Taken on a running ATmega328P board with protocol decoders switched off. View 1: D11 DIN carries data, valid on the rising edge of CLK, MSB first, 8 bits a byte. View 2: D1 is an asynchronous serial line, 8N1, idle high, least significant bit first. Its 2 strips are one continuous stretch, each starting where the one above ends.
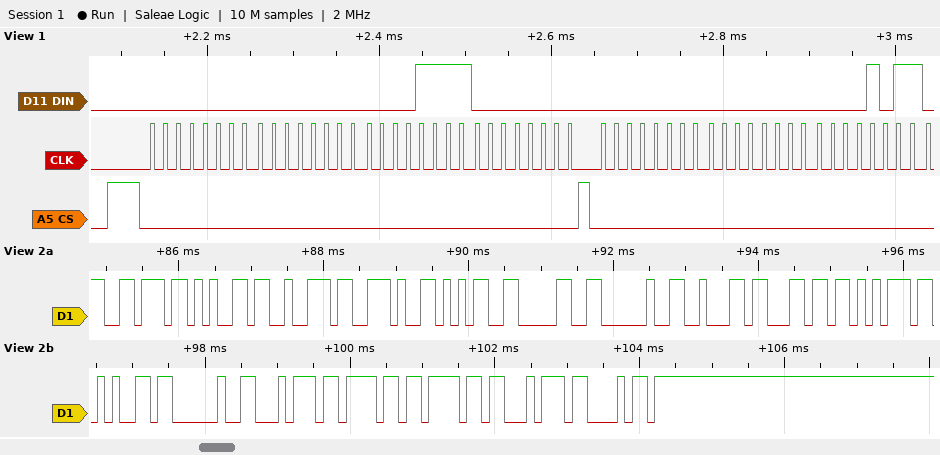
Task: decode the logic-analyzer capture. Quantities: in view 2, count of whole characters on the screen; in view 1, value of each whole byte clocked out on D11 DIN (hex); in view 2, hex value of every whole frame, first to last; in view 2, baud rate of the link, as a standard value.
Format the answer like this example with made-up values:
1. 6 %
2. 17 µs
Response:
1. 17
2. 0x00 0x00 0x0F 0x00 0x00 0x00 0x0B
3. 76 65 72 2E 35 30 20 62 6C 75 65 20 74 6F 6F 74 68
4. 9600 baud
